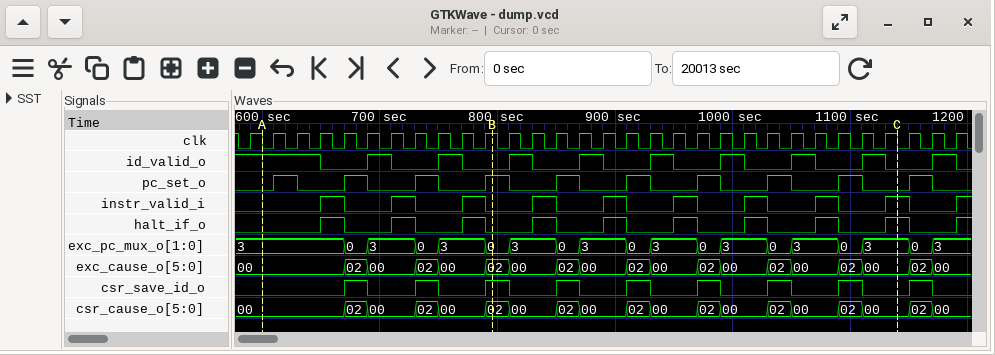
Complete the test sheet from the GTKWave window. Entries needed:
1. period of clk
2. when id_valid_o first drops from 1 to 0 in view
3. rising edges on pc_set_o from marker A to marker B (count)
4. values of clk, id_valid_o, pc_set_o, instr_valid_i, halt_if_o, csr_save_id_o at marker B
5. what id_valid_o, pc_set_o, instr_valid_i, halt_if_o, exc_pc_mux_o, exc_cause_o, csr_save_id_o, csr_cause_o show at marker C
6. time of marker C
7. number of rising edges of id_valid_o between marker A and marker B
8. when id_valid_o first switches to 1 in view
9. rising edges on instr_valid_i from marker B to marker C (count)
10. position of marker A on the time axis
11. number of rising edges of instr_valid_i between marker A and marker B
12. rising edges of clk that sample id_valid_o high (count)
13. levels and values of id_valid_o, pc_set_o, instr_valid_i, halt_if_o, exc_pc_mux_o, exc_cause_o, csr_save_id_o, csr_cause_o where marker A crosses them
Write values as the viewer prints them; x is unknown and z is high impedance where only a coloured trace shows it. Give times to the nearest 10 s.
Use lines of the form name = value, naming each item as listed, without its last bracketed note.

period of clk = 20 s
when id_valid_o first drops from 1 to 0 in view = 650 s
rising edges on pc_set_o from marker A to marker B = 4
values of clk, id_valid_o, pc_set_o, instr_valid_i, halt_if_o, csr_save_id_o at marker B = clk=1, id_valid_o=0, pc_set_o=1, instr_valid_i=0, halt_if_o=0, csr_save_id_o=1
what id_valid_o, pc_set_o, instr_valid_i, halt_if_o, exc_pc_mux_o, exc_cause_o, csr_save_id_o, csr_cause_o show at marker C = id_valid_o=0, pc_set_o=0, instr_valid_i=1, halt_if_o=1, exc_pc_mux_o=3, exc_cause_o=00, csr_save_id_o=0, csr_cause_o=00
time of marker C = 1140 s
number of rising edges of id_valid_o between marker A and marker B = 2
when id_valid_o first switches to 1 in view = 690 s
rising edges on instr_valid_i from marker B to marker C = 6
position of marker A on the time axis = 600 s
number of rising edges of instr_valid_i between marker A and marker B = 3
rising edges of clk that sample id_valid_o high = 13
levels and values of id_valid_o, pc_set_o, instr_valid_i, halt_if_o, exc_pc_mux_o, exc_cause_o, csr_save_id_o, csr_cause_o where marker A crosses them = id_valid_o=1, pc_set_o=0, instr_valid_i=0, halt_if_o=0, exc_pc_mux_o=3, exc_cause_o=00, csr_save_id_o=0, csr_cause_o=00
